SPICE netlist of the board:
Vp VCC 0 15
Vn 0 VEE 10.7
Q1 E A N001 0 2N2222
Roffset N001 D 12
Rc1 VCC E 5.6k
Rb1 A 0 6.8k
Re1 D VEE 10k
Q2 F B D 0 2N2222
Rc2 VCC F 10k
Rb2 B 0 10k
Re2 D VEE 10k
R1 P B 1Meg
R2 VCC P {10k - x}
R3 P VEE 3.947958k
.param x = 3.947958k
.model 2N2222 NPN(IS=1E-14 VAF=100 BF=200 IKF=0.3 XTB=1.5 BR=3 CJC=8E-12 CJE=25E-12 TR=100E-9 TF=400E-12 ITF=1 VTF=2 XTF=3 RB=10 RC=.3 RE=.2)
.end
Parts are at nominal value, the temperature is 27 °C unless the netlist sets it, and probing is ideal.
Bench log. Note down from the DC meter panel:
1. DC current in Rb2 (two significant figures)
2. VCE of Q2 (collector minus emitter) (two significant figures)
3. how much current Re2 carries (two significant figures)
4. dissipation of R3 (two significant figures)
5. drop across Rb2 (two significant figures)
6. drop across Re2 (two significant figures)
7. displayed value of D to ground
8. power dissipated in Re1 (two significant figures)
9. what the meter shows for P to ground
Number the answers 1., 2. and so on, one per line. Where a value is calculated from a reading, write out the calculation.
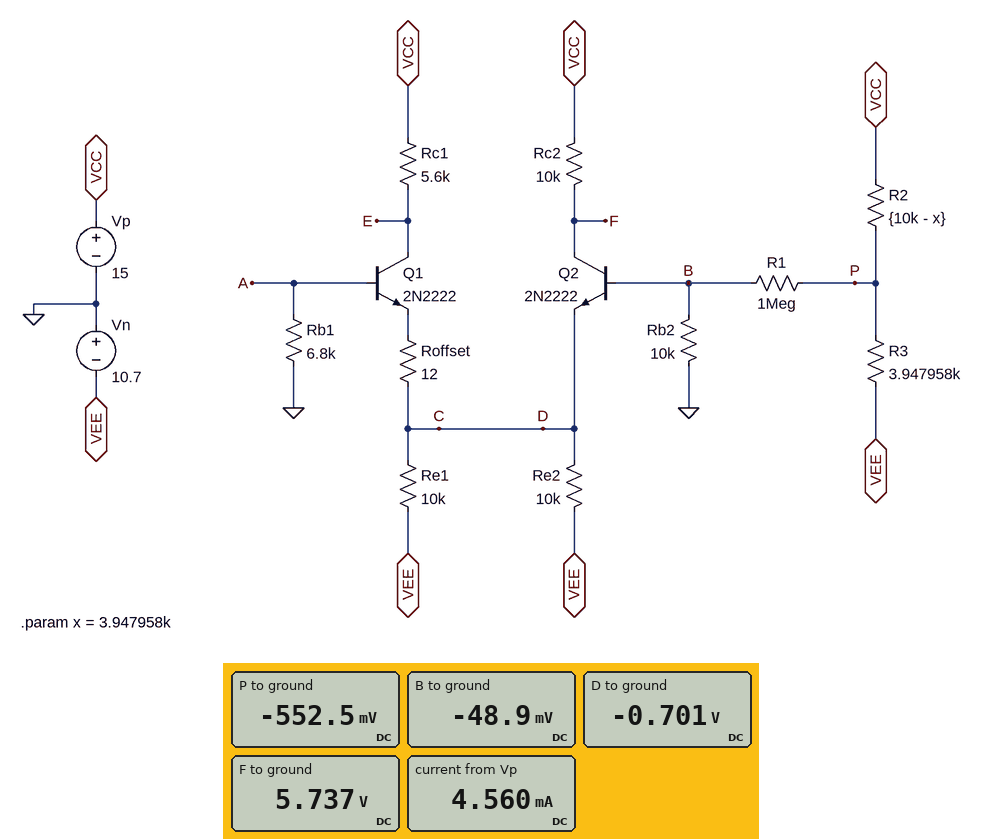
1. (0 V - (-48.9 mV)) / 10 kΩ = 4.9 µA
2. 5.737 V - (-701 mV) = 6.4 V
3. (-701 mV - (-10.7 V)) / 10 kΩ = 1.0 mA
4. (-552.5 mV - (-10.7 V))^2 / 3.948 kΩ = 26 mW
5. 0 V - (-48.9 mV) = 49 mV
6. -701 mV - (-10.7 V) = 10 V
7. -0.701 V
8. (-701 mV - (-10.7 V))^2 / 10 kΩ = 10 mW
9. -552.5 mV
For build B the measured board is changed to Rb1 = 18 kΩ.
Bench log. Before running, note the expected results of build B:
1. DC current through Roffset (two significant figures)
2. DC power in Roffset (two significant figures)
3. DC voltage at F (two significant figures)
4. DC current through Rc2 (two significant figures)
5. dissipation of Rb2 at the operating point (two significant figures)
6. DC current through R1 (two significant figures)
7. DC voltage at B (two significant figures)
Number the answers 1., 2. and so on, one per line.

1. 800 µA
2. 7.7 µW
3. 3.1 V
4. 1.2 mA
5. 390 nW
6. 490 nA
7. -63 mV
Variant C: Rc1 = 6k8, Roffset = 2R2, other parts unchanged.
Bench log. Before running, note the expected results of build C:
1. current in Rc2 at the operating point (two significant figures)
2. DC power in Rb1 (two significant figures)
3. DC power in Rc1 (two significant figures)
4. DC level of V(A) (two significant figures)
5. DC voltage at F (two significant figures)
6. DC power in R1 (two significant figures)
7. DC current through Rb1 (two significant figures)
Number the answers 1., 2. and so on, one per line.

1. 860 µA
2. 190 nW
3. 8.7 mW
4. -36 mV
5. 6.4 V
6. 260 nW
7. 5.3 µA
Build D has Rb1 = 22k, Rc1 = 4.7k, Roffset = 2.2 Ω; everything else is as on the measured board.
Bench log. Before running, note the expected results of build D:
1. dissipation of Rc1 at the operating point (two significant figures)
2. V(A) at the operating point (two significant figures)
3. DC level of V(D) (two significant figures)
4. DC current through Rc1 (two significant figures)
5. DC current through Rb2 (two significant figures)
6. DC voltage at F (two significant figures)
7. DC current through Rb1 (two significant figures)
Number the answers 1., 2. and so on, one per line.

1. 2.8 mW
2. -76 mV
3. -720 mV
4. 770 µA
5. 6.4 µA
6. 2.9 V
7. 3.5 µA
